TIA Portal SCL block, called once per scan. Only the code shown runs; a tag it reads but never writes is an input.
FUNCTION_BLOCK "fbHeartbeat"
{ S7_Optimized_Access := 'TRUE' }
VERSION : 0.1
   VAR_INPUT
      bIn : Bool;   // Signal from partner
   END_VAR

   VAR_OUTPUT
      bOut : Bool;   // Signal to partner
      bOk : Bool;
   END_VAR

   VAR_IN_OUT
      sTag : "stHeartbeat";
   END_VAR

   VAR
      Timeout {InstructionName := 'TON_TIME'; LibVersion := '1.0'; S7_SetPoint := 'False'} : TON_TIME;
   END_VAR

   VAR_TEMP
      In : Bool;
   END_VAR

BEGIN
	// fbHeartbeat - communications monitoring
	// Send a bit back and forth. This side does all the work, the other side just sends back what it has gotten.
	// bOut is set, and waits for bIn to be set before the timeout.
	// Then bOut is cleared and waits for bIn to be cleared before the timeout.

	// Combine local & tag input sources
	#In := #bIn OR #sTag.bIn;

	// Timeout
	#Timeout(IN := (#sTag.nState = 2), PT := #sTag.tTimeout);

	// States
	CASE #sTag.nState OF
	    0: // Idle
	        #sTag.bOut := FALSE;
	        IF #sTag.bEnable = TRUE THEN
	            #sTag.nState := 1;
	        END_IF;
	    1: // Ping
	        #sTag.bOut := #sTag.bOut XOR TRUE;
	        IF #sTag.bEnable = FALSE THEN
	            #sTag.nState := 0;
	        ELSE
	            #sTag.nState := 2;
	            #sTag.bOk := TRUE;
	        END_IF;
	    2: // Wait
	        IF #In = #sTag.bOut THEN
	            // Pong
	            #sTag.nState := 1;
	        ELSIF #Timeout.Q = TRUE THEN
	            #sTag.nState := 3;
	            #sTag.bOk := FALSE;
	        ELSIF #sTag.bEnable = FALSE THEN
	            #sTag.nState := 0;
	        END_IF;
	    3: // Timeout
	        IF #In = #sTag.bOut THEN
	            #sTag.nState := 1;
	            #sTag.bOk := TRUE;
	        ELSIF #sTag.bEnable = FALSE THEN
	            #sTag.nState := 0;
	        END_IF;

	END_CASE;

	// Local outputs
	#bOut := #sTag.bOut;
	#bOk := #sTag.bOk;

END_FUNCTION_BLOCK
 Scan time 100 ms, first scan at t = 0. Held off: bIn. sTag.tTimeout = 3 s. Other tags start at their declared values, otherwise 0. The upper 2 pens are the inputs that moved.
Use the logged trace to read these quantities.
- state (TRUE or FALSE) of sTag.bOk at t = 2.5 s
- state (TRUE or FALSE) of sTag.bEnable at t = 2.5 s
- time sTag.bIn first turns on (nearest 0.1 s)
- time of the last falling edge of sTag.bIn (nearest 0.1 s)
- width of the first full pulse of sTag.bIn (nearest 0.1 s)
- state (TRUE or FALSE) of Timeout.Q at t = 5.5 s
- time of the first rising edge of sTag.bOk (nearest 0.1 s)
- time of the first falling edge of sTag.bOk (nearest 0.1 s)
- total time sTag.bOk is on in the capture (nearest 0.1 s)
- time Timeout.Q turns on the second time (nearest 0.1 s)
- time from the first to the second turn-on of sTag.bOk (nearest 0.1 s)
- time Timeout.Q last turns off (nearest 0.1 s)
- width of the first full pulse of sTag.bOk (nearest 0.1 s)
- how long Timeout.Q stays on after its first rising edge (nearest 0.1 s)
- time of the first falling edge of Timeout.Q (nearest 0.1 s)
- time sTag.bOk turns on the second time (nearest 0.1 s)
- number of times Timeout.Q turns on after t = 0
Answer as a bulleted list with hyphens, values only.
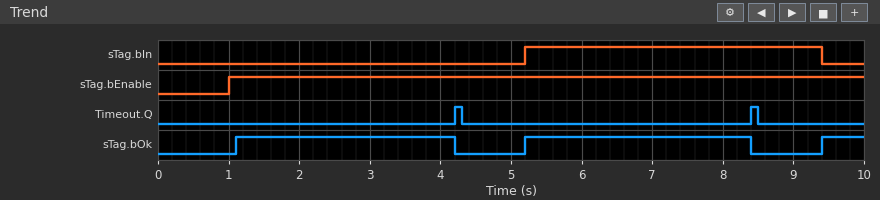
- TRUE
- TRUE
- 5.2 s
- 9.4 s
- 4.2 s
- FALSE
- 1.1 s
- 4.2 s
- 6.9 s
- 8.4 s
- 4.1 s
- 8.5 s
- 3.1 s
- 0.1 s
- 4.3 s
- 5.2 s
- 2
